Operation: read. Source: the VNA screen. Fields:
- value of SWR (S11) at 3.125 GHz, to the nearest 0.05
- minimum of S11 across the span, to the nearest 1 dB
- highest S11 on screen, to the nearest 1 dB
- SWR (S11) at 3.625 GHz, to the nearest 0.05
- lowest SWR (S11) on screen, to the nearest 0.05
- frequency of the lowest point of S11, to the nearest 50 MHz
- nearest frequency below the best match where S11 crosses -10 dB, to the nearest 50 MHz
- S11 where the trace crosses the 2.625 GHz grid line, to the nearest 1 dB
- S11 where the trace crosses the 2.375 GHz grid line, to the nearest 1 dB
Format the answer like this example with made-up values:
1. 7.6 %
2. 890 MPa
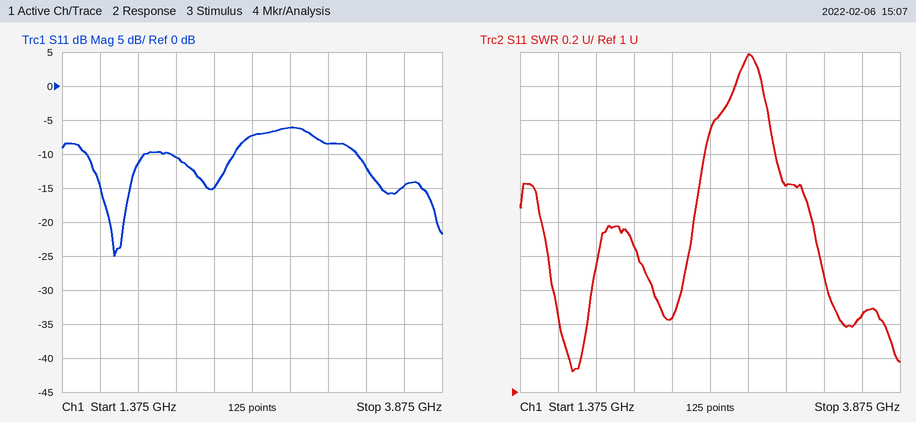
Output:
1. 2.20
2. -25 dB
3. -6 dB
4. 1.45
5. 1.10
6. 1.70 GHz
7. 1.55 GHz
8. -7 dB
9. -15 dB
